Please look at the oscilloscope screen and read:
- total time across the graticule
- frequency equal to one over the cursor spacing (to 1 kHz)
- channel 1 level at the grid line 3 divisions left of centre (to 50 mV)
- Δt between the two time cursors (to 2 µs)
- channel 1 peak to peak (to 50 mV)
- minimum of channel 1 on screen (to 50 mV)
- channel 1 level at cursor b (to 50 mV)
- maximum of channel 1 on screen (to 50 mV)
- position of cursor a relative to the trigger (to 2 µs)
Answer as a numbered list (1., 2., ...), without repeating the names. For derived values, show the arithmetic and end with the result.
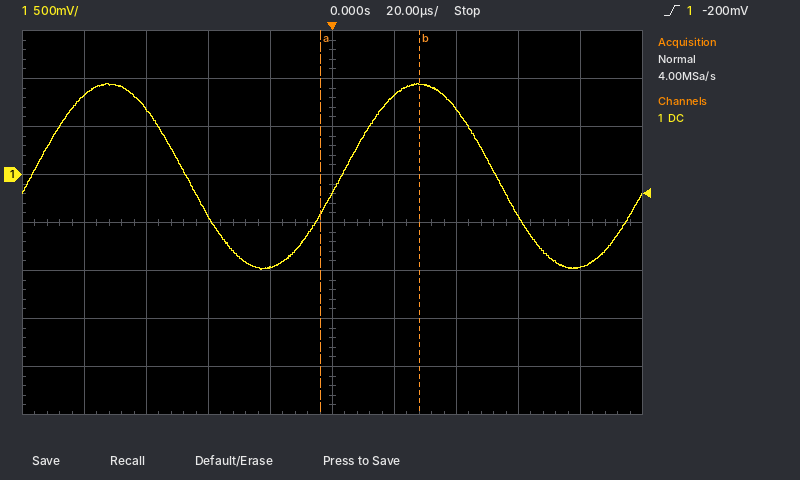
1. 200 µs
2. 1 / 32 µs ≈ 31 kHz
3. 700 mV
4. 32 µs
5. 950 mV − (-1.00 V) = 1.95 V
6. -1.00 V
7. 950 mV
8. 950 mV
9. -4 µs
